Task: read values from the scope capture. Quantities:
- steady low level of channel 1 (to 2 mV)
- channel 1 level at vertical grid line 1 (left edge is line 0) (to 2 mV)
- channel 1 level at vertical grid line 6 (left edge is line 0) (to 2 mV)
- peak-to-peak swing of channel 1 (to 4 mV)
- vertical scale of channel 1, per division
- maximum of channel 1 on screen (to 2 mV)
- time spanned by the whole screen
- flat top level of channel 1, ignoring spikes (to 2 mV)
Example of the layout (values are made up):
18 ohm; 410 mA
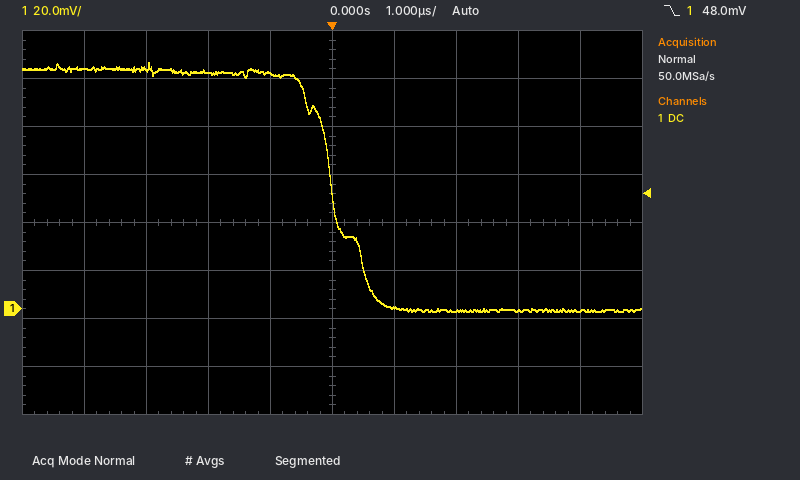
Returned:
0 mV; 100 mV; 0 mV; 104 mV; 20 mV; 102 mV; 10 µs; 100 mV
